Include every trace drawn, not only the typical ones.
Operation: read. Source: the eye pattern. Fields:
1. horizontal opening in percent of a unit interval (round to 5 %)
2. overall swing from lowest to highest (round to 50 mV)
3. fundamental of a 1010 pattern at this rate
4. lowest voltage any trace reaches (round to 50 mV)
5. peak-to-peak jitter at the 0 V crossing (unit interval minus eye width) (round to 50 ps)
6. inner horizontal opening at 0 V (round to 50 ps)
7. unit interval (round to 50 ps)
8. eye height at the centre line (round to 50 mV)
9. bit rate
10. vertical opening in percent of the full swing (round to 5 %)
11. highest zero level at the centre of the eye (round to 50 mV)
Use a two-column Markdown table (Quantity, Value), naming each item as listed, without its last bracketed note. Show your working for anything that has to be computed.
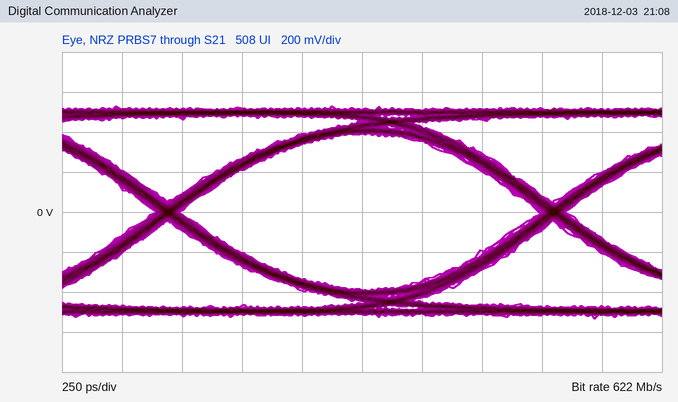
| Quantity | Value |
|---|---|
| horizontal opening in percent of a unit interval | 1.50 ns / 1.60 ns ≈ 93.7 %, so 95 % to the nearest 5 % |
| overall swing from lowest to highest | 1.05 V |
| fundamental of a 1010 pattern at this rate | 311 MHz |
| lowest voltage any trace reaches | -550 mV |
| peak-to-peak jitter at the 0 V crossing (unit interval minus eye width) | 100 ps |
| inner horizontal opening at 0 V | 1.50 ns |
| unit interval | 1.60 ns |
| eye height at the centre line | 800 mV |
| bit rate | 622 Mb/s |
| vertical opening in percent of the full swing | 800 mV / 1.05 V ≈ 76.2 %, so 75 % to the nearest 5 % |
| highest zero level at the centre of the eye | -400 mV |
